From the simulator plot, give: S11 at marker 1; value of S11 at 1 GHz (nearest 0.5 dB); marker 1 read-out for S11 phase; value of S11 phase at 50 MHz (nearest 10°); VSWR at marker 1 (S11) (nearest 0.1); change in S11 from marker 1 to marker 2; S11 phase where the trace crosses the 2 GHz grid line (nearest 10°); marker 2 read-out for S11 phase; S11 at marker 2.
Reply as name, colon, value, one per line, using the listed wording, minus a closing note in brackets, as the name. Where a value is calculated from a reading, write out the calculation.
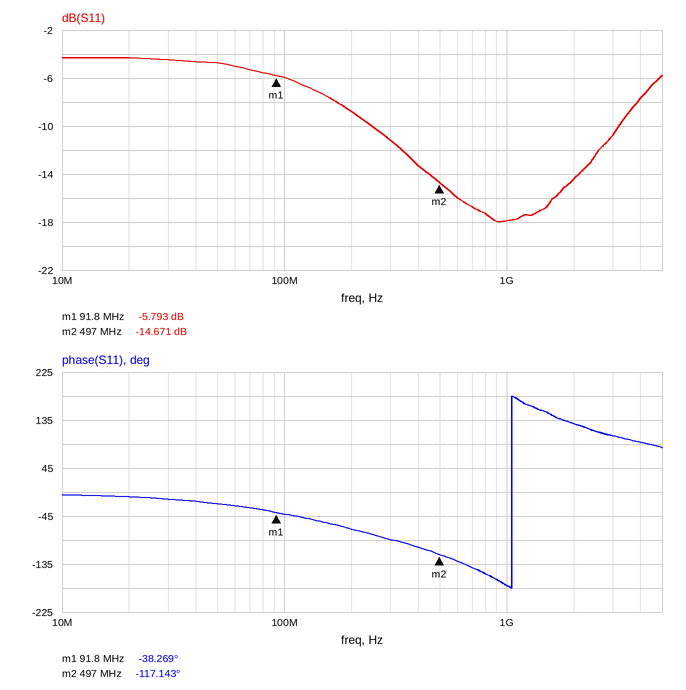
S11 at marker 1: -5.793 dB
value of S11 at 1 GHz: -18.0 dB
marker 1 read-out for S11 phase: -38.269°
value of S11 phase at 50 MHz: -20°
VSWR at marker 1 (S11): (1 + 0.5133)/(1 − 0.5133) ≈ 3.1
change in S11 from marker 1 to marker 2: -14.671 − (-5.793) = -8.878 dB
S11 phase where the trace crosses the 2 GHz grid line: 130°
marker 2 read-out for S11 phase: -117.143°
S11 at marker 2: -14.671 dB
